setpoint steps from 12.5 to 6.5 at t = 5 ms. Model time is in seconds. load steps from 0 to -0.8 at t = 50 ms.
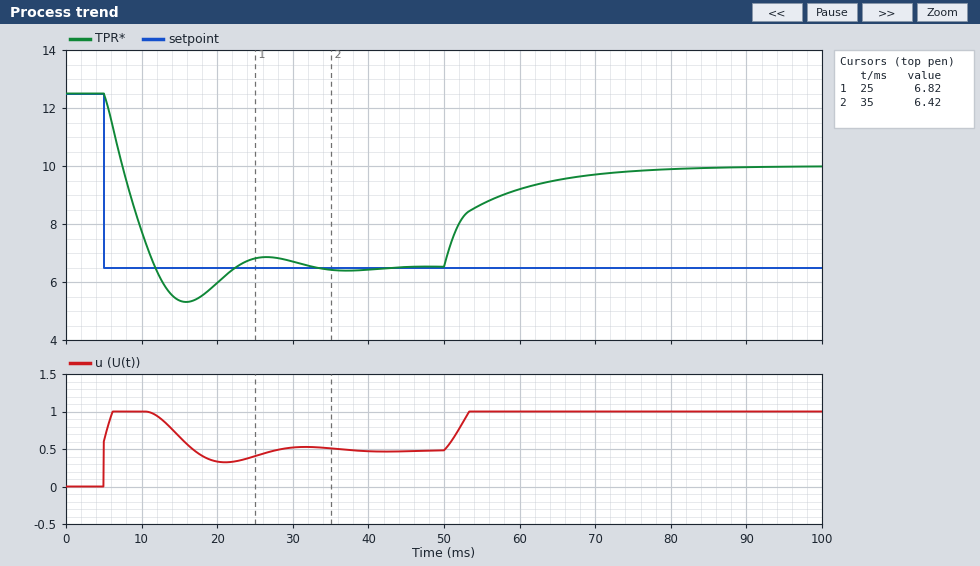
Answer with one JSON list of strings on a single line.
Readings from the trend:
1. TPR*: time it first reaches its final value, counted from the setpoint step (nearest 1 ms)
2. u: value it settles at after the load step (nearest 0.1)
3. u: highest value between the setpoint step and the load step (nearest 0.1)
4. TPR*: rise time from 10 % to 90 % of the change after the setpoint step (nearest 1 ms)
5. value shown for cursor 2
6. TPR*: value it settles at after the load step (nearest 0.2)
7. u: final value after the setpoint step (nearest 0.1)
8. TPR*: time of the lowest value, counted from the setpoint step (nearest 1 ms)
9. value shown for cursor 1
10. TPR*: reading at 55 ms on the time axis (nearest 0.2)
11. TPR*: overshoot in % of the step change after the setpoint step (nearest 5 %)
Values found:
["7 ms", "1.0", "1.0", "5 ms", "6.42", "10.0", "0.5", "11 ms", "6.82", "8.6", "20 %"]
